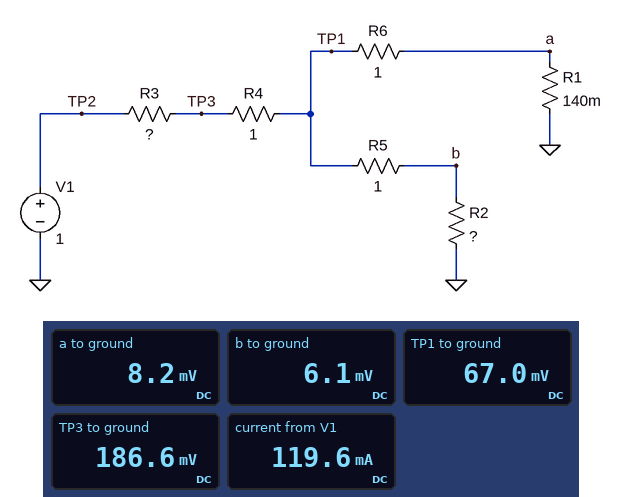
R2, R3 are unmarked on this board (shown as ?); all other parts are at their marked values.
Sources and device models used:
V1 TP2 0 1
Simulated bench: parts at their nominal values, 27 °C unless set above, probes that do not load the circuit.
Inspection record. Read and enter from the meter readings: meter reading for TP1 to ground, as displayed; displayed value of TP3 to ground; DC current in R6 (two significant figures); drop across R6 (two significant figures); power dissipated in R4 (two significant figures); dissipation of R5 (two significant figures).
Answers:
67.0 mV
186.6 mV
59 mA
59 mV
14 mW
3.7 mW
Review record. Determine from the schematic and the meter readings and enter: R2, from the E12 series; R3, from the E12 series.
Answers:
0.1 Ω
6.8 Ω
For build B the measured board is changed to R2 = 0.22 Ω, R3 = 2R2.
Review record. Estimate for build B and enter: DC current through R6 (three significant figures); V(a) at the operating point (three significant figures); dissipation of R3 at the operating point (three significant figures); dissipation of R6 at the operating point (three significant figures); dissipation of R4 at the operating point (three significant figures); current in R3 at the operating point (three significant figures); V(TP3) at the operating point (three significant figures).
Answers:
136 mA
19.1 mV
153 mW
18.6 mW
69.6 mW
264 mA
419 mV
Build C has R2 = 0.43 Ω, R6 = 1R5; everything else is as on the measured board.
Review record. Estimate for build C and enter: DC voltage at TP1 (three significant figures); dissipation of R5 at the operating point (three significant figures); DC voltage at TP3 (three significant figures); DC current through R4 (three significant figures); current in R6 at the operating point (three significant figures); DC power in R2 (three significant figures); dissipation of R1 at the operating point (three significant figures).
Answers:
89.2 mV
3.89 mW
206 mV
117 mA
54.4 mA
1.67 mW
414 µW
